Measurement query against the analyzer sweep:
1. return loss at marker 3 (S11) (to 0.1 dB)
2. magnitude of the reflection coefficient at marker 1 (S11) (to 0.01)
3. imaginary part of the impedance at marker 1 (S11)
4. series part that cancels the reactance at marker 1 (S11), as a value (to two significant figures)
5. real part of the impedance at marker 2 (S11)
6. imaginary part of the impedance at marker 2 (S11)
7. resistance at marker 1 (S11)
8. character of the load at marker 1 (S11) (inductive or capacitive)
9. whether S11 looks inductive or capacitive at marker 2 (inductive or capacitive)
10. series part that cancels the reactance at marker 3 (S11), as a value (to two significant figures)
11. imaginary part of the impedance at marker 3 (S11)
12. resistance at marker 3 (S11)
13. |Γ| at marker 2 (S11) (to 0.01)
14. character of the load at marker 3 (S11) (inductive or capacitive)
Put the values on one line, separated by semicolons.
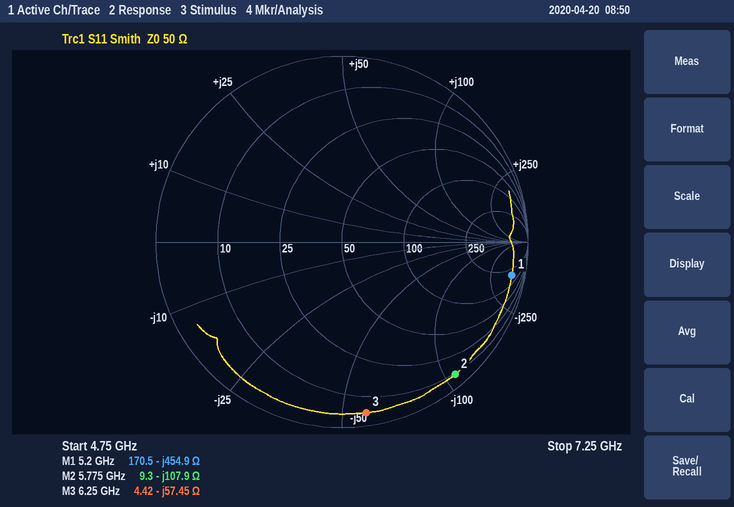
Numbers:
0.7 dB; 0.93; -454.9 Ω; 14 nH; 9.3 Ω; -107.9 Ω; 170.5 Ω; capacitive; capacitive; 1.5 nH; -57.45 Ω; 4.42 Ω; 0.94; capacitive
